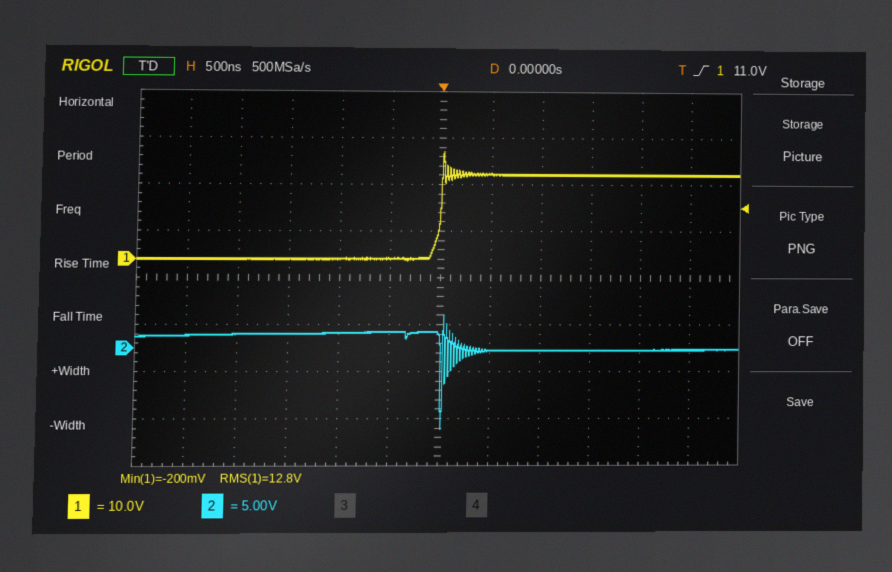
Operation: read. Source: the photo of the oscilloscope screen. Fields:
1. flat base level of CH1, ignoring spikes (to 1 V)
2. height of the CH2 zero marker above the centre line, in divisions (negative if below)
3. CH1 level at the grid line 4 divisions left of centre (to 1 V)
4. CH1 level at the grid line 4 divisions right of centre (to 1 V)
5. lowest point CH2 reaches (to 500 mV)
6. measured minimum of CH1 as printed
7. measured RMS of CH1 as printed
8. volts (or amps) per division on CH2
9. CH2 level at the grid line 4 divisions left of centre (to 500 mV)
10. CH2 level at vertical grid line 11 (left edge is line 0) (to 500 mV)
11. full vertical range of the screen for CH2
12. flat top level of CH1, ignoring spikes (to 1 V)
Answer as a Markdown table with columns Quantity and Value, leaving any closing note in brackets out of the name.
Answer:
| Quantity | Value |
|---|---|
| flat base level of CH1, ignoring spikes | 0 V |
| height of the CH2 zero marker above the centre line, in divisions | -1.5 div |
| CH1 level at the grid line 4 divisions left of centre | 0 V |
| CH1 level at the grid line 4 divisions right of centre | 18 V |
| lowest point CH2 reaches | -8.5 V |
| measured minimum of CH1 as printed | -200 mV |
| measured RMS of CH1 as printed | 12.8 V |
| volts (or amps) per division on CH2 | 5 V |
| CH2 level at the grid line 4 divisions left of centre | 1.5 V |
| CH2 level at vertical grid line 11 (left edge is line 0) | 0.0 V |
| full vertical range of the screen for CH2 | 40 V |
| flat top level of CH1, ignoring spikes | 18 V |
